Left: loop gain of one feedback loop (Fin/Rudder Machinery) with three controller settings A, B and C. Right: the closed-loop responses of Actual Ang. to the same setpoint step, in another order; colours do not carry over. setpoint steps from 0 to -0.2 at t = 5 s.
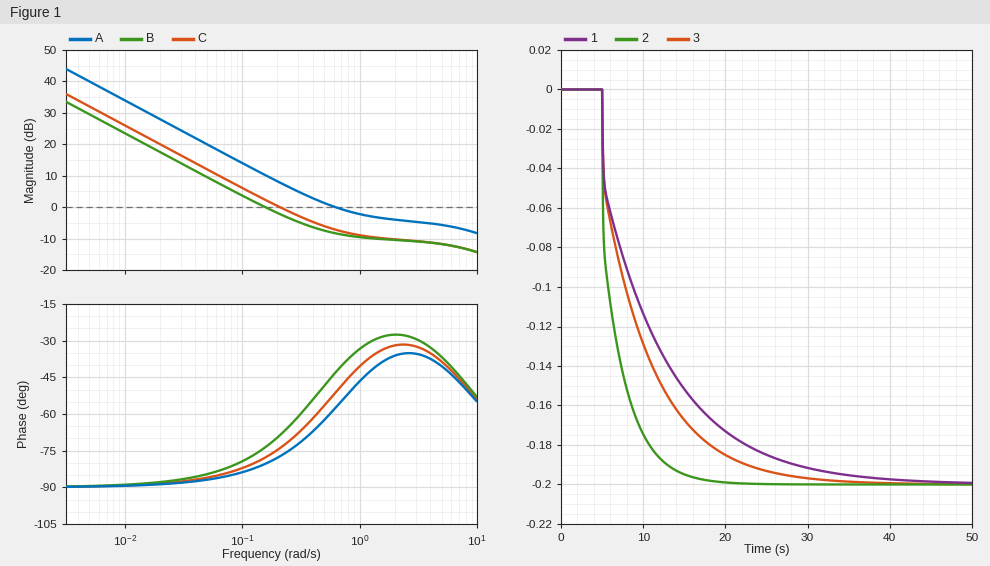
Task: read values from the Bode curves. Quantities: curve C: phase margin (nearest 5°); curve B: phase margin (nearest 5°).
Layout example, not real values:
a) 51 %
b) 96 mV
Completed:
a) 105°
b) 105°
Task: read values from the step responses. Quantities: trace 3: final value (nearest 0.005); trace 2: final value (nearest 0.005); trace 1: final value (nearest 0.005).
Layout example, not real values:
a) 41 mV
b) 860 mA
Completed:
a) -0.200
b) -0.200
c) -0.200
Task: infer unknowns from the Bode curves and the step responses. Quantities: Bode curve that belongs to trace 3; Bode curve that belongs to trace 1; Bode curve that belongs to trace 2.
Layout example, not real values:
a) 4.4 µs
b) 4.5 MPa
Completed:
a) C
b) B
c) A
